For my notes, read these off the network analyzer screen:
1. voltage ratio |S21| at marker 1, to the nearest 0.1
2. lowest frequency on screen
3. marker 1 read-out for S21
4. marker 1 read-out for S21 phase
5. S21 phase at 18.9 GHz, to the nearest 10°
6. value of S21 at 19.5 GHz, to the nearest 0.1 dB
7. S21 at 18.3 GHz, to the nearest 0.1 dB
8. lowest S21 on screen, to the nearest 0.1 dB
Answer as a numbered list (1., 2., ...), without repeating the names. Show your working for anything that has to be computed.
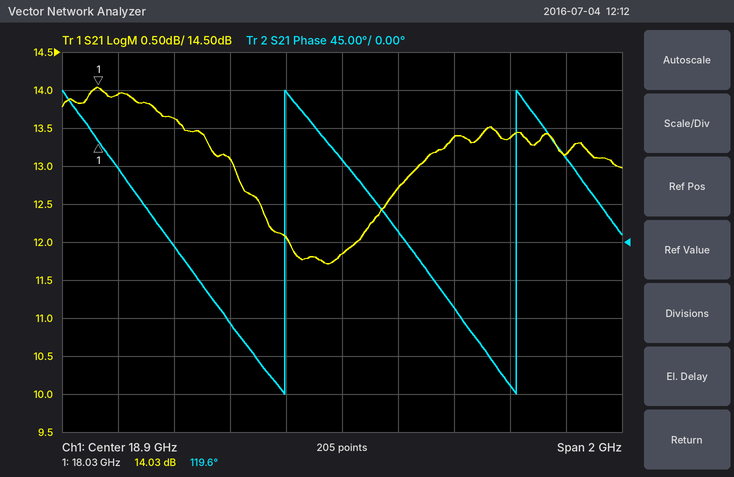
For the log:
1. 10^(14.03/20) ≈ 5.0
2. 17.9 GHz
3. 14.03 dB
4. 119.6°
5. 100°
6. 13.4 dB
7. 13.6 dB
8. 11.7 dB
